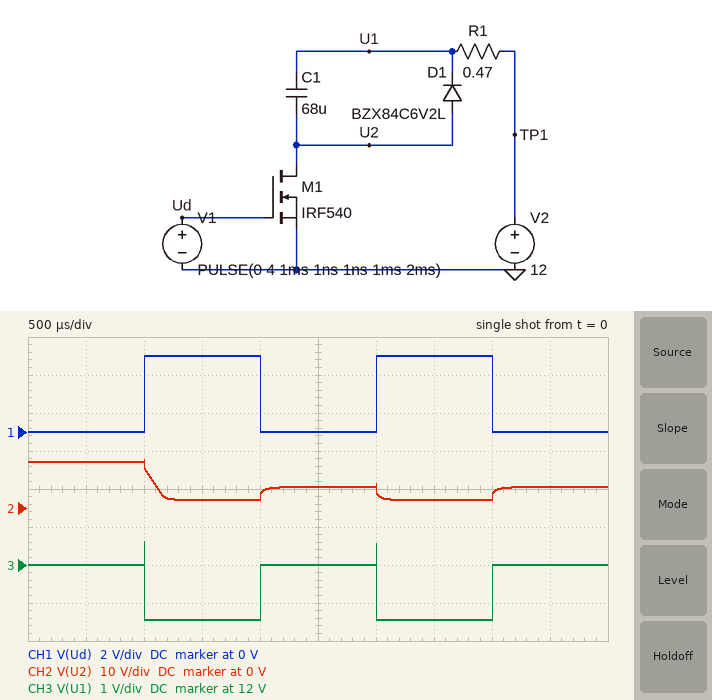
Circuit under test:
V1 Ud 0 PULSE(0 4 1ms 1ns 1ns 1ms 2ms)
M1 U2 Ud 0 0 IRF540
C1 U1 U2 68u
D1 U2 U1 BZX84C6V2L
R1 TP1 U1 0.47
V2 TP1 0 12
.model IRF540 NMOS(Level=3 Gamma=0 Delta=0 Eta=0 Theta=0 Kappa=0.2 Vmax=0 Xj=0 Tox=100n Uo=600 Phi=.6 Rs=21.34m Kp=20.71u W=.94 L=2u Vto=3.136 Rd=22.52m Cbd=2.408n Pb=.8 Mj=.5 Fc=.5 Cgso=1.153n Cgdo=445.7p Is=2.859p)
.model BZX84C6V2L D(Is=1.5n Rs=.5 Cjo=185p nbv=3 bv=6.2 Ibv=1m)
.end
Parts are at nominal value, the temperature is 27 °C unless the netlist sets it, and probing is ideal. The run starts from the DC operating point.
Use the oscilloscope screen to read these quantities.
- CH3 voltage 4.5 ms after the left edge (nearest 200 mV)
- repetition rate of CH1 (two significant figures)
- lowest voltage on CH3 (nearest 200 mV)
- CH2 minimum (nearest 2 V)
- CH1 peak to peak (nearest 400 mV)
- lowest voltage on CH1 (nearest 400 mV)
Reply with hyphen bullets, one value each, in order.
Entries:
- 12.0 V
- 500 Hz
- 10.6 V
- 2 V
- 4.0 V
- 0 V
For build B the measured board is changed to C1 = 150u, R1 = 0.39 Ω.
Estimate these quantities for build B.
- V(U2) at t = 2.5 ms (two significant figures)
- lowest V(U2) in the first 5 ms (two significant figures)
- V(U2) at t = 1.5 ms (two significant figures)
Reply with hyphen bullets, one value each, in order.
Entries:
- 5.5 V
- 2.4 V
- 2.6 V
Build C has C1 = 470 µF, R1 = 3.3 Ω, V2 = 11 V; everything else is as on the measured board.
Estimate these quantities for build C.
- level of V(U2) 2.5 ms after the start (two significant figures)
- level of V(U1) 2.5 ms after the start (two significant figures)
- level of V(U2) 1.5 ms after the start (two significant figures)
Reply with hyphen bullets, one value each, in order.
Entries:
- 6.0 V
- 11 V
- 480 mV
